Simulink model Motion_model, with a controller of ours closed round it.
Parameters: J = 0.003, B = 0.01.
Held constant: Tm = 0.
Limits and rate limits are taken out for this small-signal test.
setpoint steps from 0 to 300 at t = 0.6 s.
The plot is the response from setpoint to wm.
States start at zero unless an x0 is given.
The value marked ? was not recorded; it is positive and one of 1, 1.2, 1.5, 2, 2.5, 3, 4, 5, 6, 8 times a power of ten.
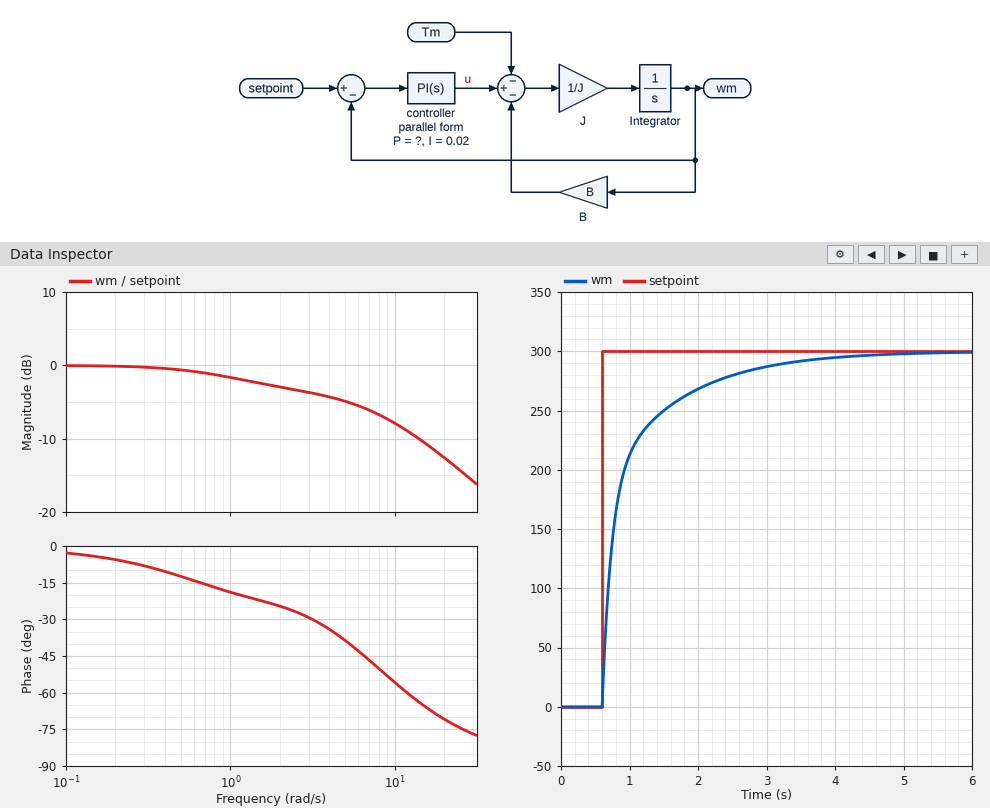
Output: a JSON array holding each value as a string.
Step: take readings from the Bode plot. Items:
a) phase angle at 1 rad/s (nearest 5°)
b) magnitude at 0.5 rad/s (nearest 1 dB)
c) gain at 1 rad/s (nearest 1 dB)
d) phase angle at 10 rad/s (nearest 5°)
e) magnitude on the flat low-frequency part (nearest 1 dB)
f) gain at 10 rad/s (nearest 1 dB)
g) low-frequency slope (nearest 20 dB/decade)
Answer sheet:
["-20°", "-1 dB", "-2 dB", "-55°", "0 dB", "-8 dB", "0 dB/decade"]
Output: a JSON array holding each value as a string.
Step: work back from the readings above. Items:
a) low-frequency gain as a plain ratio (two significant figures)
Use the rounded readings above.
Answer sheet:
["1.0"]
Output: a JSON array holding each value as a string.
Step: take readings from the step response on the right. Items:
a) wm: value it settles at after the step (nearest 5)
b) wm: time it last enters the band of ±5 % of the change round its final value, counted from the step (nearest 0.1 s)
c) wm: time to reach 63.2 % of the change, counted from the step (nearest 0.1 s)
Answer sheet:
["300", "2.2 s", "0.3 s"]
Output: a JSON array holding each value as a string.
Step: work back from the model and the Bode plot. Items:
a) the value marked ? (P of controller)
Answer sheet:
["0.015"]
